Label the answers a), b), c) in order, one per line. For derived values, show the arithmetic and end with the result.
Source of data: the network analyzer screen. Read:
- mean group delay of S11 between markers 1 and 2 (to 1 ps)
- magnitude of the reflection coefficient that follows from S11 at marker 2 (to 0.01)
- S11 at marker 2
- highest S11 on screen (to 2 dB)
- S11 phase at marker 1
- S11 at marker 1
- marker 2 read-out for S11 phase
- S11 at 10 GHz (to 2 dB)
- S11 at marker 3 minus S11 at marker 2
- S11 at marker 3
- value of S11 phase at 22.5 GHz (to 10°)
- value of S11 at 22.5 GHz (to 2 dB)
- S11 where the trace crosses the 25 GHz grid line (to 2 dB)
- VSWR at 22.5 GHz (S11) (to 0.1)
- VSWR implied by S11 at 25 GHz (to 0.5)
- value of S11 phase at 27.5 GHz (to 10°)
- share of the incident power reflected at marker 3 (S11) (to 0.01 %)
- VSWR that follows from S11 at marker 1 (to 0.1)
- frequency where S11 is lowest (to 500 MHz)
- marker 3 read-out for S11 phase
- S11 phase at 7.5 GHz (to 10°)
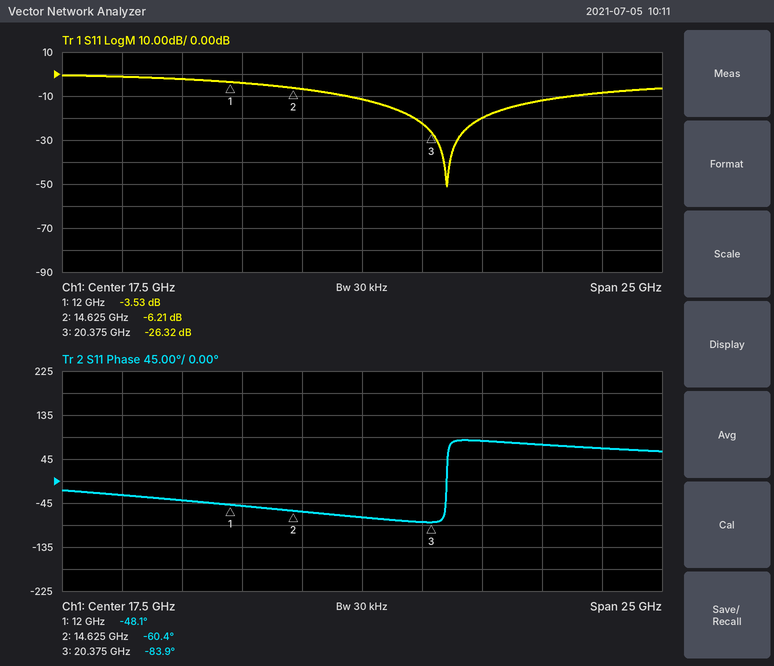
a) −(-60.4° − (-48.1°))/(360° × 2.625 GHz) ≈ 13 ps
b) 10^(-6.21/20) ≈ 0.49
c) -6.21 dB
d) 0 dB
e) -48.1°
f) -3.53 dB
g) -60.4°
h) -2 dB
i) -26.32 − (-6.21) = -20.11 dB
j) -26.32 dB
k) 80°
l) -20 dB
m) -12 dB
n) |Γ| = 10^(-20/20) = 0.1000; VSWR = (1 + 0.1000)/(1 − 0.1000) ≈ 1.2
o) |Γ| = 10^(-12/20) = 0.2512; VSWR = (1 + 0.2512)/(1 − 0.2512) ≈ 1.67, so 1.5 to the nearest 0.5
p) 70°
q) 10^(-26.32/10) ≈ 0.23 %
r) (1 + 0.6660)/(1 − 0.6660) ≈ 5.0
s) 21.0 GHz
t) -83.9°
u) -30°
